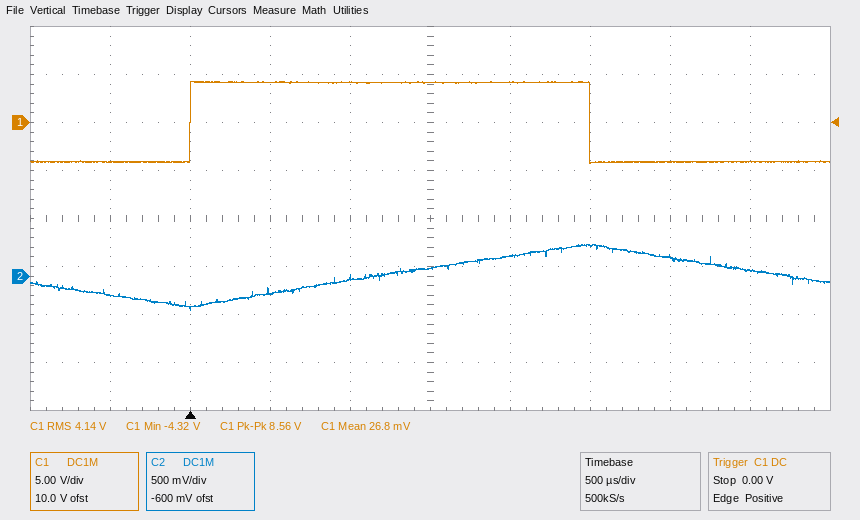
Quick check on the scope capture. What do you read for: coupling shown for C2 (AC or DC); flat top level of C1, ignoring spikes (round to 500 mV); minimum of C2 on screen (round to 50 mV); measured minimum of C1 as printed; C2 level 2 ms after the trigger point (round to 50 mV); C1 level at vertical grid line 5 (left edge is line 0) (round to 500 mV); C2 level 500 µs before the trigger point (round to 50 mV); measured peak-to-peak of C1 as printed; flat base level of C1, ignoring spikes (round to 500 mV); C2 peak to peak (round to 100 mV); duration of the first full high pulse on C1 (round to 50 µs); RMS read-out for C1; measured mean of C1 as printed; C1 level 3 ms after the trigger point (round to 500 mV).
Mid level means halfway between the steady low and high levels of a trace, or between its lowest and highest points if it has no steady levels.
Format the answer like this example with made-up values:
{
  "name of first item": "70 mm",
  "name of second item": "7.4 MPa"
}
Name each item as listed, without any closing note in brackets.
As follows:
{
  "coupling shown for C2": "DC",
  "flat top level of C1, ignoring spikes": "4.0 V",
  "minimum of C2 on screen": "-350 mV",
  "measured minimum of C1 as printed": "-4.32 V",
  "C2 level 2 ms after the trigger point": "200 mV",
  "C1 level at vertical grid line 5 (left edge is line 0)": "4.0 V",
  "C2 level 500 µs before the trigger point": "-200 mV",
  "measured peak-to-peak of C1 as printed": "8.56 V",
  "flat base level of C1, ignoring spikes": "-4.0 V",
  "C2 peak to peak": "700 mV",
  "duration of the first full high pulse on C1": "2.50 ms",
  "RMS read-out for C1": "4.14 V",
  "measured mean of C1 as printed": "26.8 mV",
  "C1 level 3 ms after the trigger point": "-4.0 V"
}
